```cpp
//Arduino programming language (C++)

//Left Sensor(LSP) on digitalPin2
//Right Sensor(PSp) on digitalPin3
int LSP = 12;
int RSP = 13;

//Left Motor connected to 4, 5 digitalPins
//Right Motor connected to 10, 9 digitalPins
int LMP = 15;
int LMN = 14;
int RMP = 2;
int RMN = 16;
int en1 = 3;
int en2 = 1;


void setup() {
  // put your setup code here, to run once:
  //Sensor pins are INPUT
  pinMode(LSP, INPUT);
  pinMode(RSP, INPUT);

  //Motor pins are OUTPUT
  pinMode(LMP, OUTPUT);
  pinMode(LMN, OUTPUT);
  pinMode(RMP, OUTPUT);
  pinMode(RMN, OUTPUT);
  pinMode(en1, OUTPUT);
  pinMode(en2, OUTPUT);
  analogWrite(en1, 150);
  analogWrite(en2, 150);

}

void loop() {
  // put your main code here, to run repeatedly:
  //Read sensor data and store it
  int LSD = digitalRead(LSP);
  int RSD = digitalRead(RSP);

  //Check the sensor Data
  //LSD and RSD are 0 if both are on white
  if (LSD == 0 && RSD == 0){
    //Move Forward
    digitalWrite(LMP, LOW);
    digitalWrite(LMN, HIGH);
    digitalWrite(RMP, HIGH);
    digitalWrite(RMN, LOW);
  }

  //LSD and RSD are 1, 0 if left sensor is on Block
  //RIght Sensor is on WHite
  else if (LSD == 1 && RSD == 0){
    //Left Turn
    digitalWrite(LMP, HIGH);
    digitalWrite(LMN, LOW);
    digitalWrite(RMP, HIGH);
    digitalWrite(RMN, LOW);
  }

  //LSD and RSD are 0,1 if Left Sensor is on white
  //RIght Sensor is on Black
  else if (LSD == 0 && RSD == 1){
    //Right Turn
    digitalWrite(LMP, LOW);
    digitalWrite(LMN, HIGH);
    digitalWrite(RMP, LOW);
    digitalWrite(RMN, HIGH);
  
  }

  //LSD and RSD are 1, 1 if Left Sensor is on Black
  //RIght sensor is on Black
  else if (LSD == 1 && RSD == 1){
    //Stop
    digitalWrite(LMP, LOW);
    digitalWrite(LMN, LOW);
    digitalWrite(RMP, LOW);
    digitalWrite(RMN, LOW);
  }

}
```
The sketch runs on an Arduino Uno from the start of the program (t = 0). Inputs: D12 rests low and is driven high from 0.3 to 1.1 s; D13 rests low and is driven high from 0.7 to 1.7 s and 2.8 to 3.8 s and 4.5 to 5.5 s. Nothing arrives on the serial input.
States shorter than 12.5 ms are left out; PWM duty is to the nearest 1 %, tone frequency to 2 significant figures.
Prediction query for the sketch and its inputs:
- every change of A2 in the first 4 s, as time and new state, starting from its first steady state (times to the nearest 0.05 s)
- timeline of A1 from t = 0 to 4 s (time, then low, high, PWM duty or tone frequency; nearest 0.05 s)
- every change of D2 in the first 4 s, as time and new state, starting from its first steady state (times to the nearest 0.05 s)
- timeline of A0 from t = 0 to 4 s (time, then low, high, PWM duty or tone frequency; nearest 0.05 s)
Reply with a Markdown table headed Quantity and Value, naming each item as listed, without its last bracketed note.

| Quantity | Value |
|---|---|
| every change of A2 in the first 4 s, as time and new state, starting from its first steady state | 0 s low; 1.1 s high; 1.7 s low; 2.8 s high; 3.8 s low |
| timeline of A1 from t = 0 to 4 s | 0 s low; 0.3 s high; 0.7 s low |
| every change of D2 in the first 4 s, as time and new state, starting from its first steady state | 0 s high; 0.7 s low; 1.7 s high; 2.8 s low; 3.8 s high |
| timeline of A0 from t = 0 to 4 s | 0 s high; 0.3 s low; 1.1 s high |
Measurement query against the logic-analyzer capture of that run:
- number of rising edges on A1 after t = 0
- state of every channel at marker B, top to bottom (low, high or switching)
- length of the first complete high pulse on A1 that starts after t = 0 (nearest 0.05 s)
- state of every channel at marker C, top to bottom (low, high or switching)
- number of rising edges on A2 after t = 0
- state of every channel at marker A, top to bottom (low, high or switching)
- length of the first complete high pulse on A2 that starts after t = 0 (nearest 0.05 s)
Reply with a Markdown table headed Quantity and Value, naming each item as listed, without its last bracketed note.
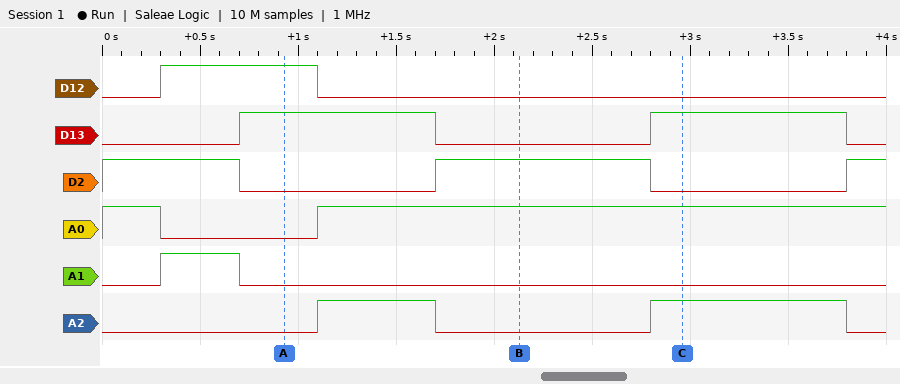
| Quantity | Value |
|---|---|
| number of rising edges on A1 after t = 0 | 1 |
| state of every channel at marker B, top to bottom | D12 low, D13 low, D2 high, A0 high, A1 low, A2 low |
| length of the first complete high pulse on A1 that starts after t = 0 | 0.40 s |
| state of every channel at marker C, top to bottom | D12 low, D13 high, D2 low, A0 high, A1 low, A2 high |
| number of rising edges on A2 after t = 0 | 2 |
| state of every channel at marker A, top to bottom | D12 high, D13 high, D2 low, A0 low, A1 low, A2 low |
| length of the first complete high pulse on A2 that starts after t = 0 | 0.60 s |
